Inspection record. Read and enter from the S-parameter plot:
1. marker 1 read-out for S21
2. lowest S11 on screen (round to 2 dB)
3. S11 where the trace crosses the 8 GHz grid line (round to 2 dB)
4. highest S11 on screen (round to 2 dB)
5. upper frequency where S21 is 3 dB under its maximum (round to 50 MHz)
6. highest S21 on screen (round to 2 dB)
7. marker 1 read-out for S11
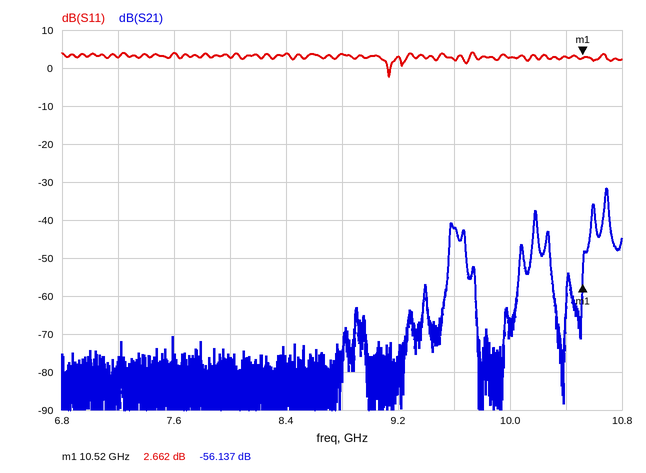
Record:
-56.137 dB
-2 dB
2 dB
4 dB
10.70 GHz
-32 dB
2.662 dB
